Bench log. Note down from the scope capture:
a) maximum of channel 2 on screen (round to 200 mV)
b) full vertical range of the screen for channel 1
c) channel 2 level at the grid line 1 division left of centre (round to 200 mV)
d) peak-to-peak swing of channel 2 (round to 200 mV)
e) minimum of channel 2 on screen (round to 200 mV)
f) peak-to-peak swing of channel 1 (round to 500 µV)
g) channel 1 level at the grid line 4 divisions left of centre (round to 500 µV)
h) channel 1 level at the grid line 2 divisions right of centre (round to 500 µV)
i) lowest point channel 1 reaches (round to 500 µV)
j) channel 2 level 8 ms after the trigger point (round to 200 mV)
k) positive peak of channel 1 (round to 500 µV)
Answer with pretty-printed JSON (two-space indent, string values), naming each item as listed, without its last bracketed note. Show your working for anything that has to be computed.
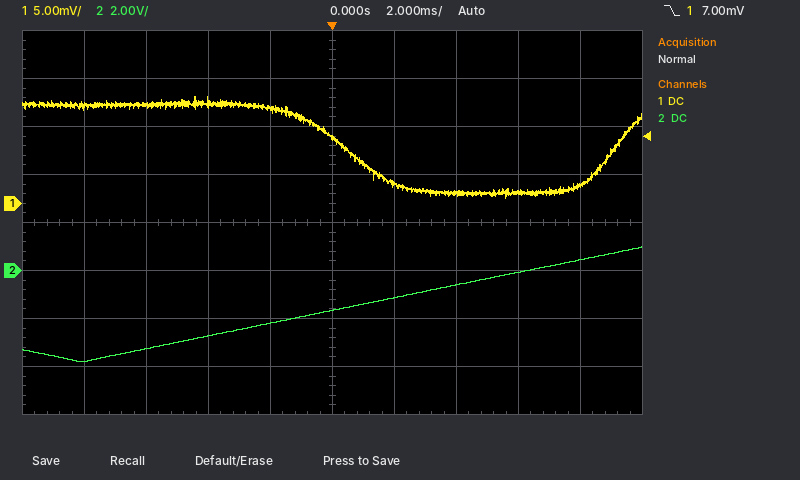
{
  "maximum of channel 2 on screen": "1.0 V",
  "full vertical range of the screen for channel 1": "40 mV",
  "channel 2 level at the grid line 1 division left of centre": "-2.2 V",
  "peak-to-peak swing of channel 2": "1.0 V − (-3.8 V) = 4.8 V",
  "minimum of channel 2 on screen": "-3.8 V",
  "peak-to-peak swing of channel 1": "11.0 mV − (500 µV) = 10.5 mV",
  "channel 1 level at the grid line 4 divisions left of centre": "10.0 mV",
  "channel 1 level at the grid line 2 divisions right of centre": "1.0 mV",
  "lowest point channel 1 reaches": "500 µV",
  "channel 2 level 8 ms after the trigger point": "400 mV",
  "positive peak of channel 1": "11.0 mV"
}
